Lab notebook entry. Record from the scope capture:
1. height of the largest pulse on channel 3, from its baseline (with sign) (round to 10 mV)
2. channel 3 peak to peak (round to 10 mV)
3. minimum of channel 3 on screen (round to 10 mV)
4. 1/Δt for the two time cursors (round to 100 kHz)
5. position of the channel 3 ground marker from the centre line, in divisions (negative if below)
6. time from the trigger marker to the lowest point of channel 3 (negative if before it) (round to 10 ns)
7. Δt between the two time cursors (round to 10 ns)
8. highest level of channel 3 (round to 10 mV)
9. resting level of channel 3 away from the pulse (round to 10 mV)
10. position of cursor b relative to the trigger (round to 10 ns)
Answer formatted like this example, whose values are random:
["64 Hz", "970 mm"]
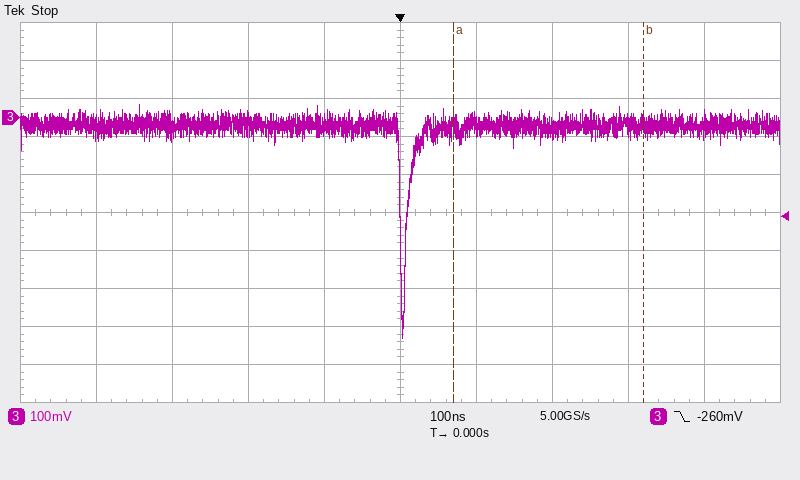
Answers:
["-560 mV", "610 mV", "-580 mV", "4.0 MHz", "+2.5 div", "0 ns", "250 ns", "30 mV", "-20 mV", "+320 ns"]
